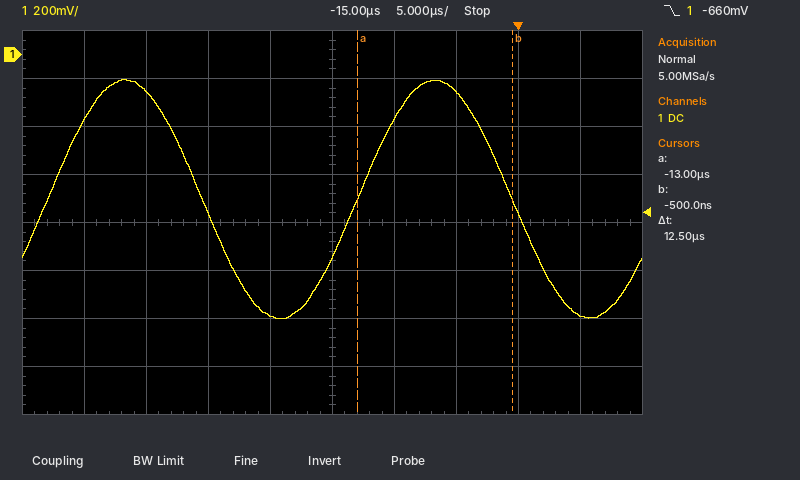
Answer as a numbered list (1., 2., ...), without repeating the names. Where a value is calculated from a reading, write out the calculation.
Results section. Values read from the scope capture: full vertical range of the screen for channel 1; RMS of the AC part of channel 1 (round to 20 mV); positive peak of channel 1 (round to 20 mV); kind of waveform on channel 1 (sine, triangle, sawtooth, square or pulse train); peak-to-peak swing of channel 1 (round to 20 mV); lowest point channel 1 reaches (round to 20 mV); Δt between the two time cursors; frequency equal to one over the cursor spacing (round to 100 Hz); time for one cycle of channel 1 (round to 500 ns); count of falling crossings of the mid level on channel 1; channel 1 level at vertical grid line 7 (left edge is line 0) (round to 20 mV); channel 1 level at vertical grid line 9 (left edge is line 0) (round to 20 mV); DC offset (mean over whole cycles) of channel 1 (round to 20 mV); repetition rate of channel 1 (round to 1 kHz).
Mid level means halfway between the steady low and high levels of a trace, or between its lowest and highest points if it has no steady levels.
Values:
1. 1.6 V
2. 1.00 V / (2√2) ≈ 354 mV, so 360 mV to the nearest 20 mV
3. -100 mV
4. sine
5. -100 mV − (-1.10 V) = 1.00 V
6. -1.10 V
7. 12.5 µs
8. 1 / 12.5 µs ≈ 80.0 kHz
9. 25.0 µs
10. 2
11. -160 mV
12. -1.08 V
13. (-100 mV + (-1.10 V)) / 2 ≈ -600 mV
14. 1 / 25.0 µs ≈ 40 kHz
